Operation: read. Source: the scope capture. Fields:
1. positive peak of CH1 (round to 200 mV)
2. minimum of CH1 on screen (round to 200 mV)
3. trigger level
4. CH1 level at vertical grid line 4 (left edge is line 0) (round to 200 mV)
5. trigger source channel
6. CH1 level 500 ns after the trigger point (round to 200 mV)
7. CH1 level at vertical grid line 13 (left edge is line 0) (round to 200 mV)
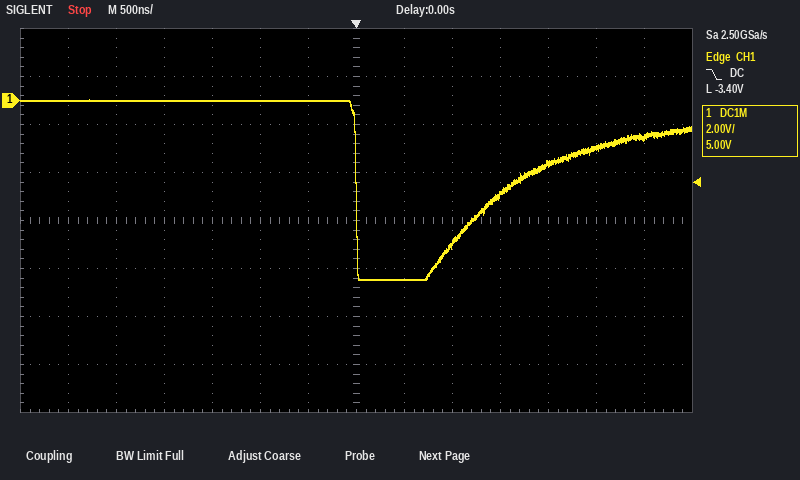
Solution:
0.0 V
-7.4 V
-3.40 V
0.0 V
CH1
-7.4 V
-1.6 V
